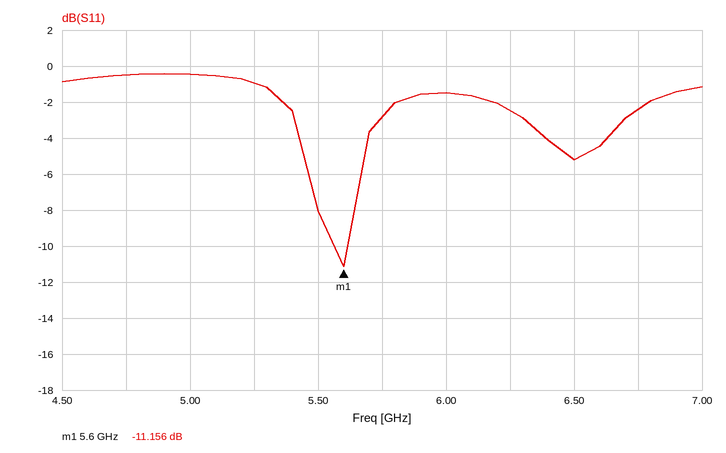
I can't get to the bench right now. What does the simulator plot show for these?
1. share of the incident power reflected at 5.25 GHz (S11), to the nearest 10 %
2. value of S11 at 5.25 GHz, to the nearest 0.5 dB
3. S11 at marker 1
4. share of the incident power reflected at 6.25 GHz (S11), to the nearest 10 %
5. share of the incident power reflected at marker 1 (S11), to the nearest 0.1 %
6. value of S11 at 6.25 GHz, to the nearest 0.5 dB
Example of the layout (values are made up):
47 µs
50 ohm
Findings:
80 %
-1.0 dB
-11.156 dB
60 %
7.7 %
-2.5 dB
